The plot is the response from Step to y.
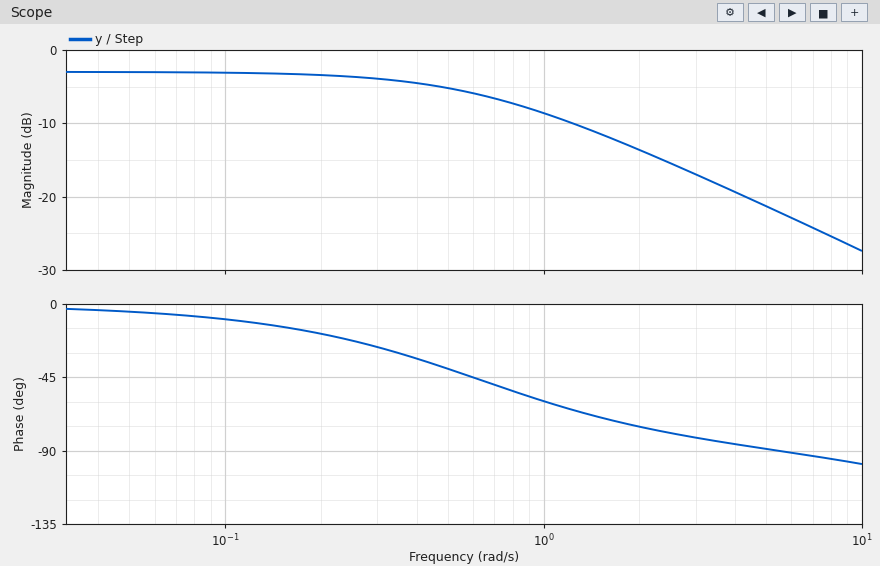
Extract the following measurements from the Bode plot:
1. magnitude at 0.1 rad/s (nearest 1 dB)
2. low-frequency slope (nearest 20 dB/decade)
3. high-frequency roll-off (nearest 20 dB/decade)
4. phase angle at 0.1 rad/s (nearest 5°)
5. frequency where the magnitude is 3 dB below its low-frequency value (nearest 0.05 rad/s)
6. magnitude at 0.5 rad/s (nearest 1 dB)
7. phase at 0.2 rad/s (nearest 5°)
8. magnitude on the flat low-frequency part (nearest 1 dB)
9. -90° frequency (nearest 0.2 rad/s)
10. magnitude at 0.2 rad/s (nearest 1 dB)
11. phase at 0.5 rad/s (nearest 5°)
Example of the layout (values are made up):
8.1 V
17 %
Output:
-3 dB
0 dB/decade
-20 dB/decade
-10°
0.60 rad/s
-5 dB
-20°
-3 dB
5.4 rad/s
-3 dB
-40°
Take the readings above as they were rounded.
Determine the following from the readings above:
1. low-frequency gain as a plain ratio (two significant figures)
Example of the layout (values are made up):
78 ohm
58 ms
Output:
0.71
